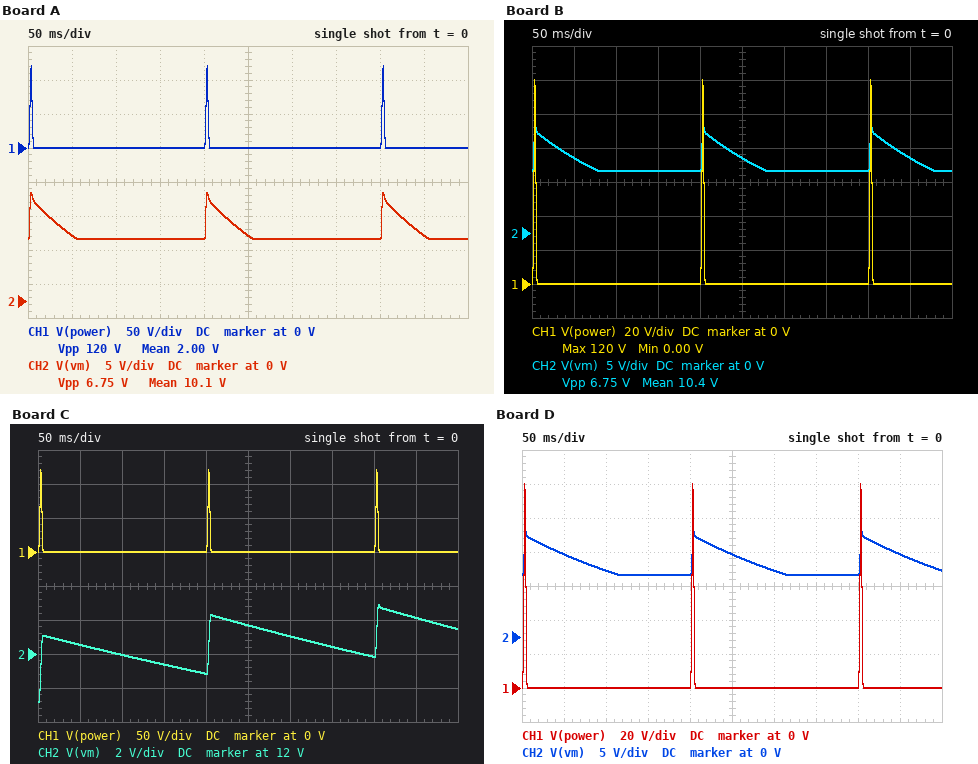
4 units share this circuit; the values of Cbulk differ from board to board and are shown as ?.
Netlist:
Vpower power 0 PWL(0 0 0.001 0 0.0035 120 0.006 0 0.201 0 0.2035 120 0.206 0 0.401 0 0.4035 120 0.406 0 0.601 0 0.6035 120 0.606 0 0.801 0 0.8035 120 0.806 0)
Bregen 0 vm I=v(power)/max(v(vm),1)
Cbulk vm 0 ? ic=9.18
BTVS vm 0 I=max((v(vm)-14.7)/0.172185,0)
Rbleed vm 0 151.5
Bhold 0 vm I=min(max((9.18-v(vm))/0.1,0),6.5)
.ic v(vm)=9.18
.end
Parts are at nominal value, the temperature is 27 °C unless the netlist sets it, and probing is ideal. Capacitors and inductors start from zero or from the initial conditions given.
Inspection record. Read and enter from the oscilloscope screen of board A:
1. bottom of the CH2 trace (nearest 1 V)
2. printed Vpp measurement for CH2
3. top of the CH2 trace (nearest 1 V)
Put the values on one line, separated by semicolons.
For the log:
9 V; 6.75 V; 16 V
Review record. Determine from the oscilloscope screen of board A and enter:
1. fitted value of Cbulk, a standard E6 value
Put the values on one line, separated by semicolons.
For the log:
680 µF
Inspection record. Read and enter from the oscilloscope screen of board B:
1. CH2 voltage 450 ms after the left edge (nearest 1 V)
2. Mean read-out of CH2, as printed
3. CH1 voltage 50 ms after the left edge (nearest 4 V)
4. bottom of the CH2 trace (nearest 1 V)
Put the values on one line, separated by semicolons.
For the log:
11 V; 10.4 V; 0 V; 9 V
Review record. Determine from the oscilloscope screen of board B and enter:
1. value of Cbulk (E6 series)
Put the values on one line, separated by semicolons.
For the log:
1 mF
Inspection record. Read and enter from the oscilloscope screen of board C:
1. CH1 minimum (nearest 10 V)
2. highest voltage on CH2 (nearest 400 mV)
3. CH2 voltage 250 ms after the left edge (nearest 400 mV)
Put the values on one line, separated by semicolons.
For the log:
0 V; 14.8 V; 13.6 V
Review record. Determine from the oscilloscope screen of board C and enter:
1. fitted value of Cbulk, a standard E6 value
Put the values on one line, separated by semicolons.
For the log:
6.8 mF
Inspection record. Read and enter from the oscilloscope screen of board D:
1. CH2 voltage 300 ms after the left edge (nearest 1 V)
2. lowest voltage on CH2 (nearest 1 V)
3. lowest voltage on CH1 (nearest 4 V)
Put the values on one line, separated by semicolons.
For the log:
10 V; 9 V; 0 V
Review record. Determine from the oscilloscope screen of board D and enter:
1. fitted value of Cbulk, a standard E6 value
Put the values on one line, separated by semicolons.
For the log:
1.5 mF
